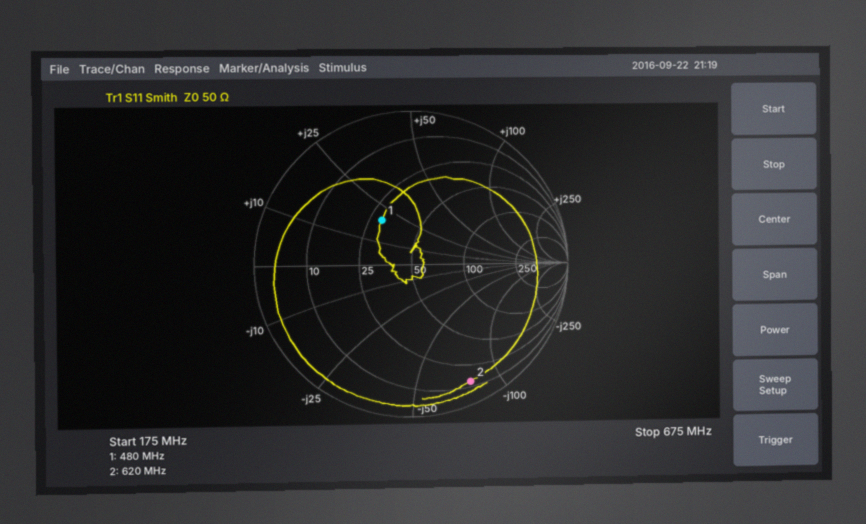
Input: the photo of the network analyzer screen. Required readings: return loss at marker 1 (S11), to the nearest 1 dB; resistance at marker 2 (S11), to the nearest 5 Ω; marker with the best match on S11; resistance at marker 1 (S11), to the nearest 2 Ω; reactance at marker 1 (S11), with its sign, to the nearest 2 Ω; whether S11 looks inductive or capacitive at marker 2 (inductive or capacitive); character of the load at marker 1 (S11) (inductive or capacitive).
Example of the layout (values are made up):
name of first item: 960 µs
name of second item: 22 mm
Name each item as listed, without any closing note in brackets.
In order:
return loss at marker 1 (S11), to the nearest 1 dB: 9 dB
resistance at marker 2 (S11), to the nearest 5 Ω: 15 Ω
marker with the best match on S11: marker 1
resistance at marker 1 (S11), to the nearest 2 Ω: 30 Ω
reactance at marker 1 (S11), with its sign, to the nearest 2 Ω: +20 Ω
whether S11 looks inductive or capacitive at marker 2: capacitive
character of the load at marker 1 (S11): inductive
